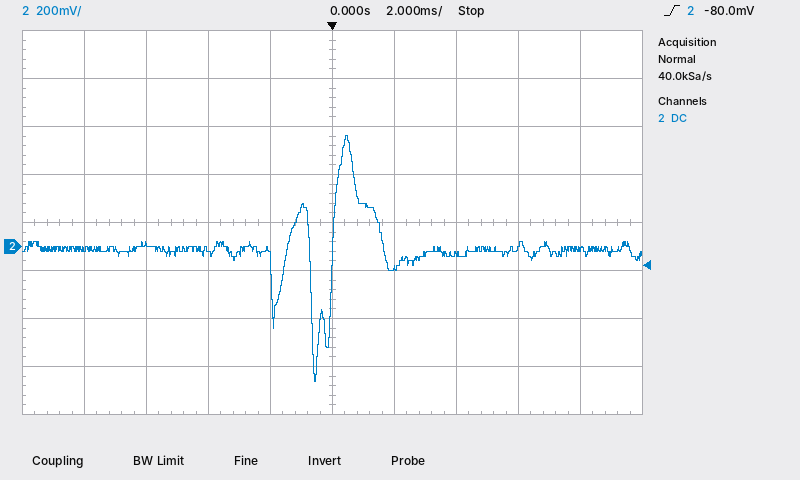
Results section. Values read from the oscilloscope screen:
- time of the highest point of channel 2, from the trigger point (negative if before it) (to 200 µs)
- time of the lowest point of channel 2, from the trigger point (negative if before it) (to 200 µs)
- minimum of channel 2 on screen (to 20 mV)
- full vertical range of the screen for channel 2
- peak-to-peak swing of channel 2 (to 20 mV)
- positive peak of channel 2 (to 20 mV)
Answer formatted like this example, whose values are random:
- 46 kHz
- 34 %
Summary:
- +400 µs
- -600 µs
- -560 mV
- 1.6 V
- 1.02 V
- 460 mV
